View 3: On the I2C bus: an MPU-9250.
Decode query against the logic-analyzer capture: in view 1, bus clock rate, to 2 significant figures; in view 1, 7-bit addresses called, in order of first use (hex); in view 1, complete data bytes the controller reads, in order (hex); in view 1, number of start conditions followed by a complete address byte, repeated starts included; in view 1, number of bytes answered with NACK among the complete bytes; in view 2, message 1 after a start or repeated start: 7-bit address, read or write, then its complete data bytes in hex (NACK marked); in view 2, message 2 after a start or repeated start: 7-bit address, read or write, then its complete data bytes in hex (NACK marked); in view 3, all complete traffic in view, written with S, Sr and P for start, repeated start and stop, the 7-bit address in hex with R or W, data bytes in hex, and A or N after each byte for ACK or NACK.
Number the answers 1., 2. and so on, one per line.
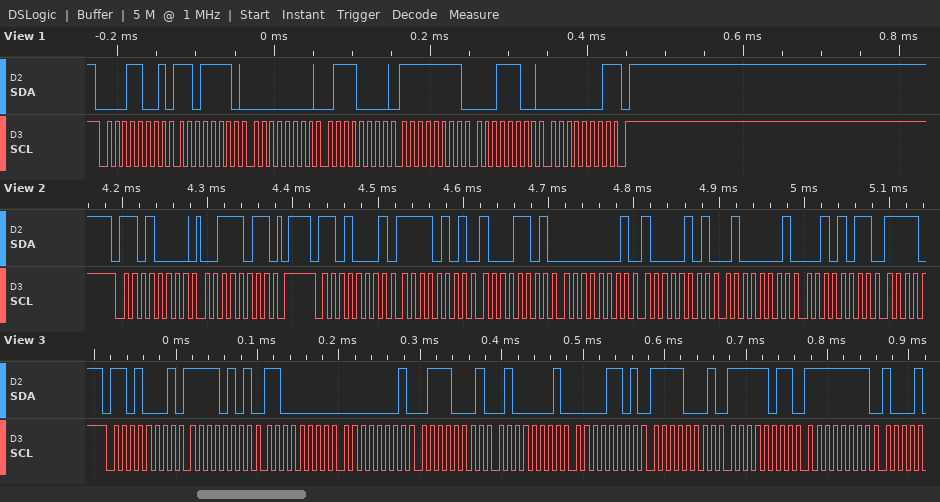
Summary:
1. 100 kHz
2. 0x0C
3. DE 00 70 FF 1C 01
4. 1
5. 1
6. 0x68 write: 3B
7. 0x68 read: F5 8D 01 85 41 2B
8. S 68R A F5 A C0 A 01 A 71 A 41 A 0D A F1 A FB A FF A
